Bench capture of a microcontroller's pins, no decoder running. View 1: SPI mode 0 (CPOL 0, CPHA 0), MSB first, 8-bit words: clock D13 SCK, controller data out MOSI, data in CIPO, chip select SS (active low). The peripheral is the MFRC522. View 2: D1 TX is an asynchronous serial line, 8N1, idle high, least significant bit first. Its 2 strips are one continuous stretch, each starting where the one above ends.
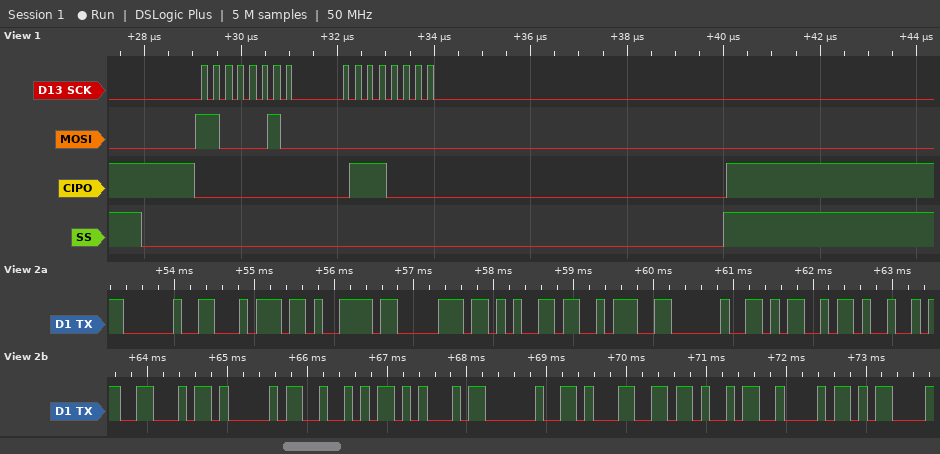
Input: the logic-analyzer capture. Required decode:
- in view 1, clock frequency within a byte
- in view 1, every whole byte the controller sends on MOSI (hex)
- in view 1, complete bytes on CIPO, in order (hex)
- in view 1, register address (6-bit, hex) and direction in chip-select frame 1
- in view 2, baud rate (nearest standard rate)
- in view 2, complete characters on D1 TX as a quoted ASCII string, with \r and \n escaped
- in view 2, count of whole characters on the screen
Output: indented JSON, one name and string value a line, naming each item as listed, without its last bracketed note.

{
  "in view 1, clock frequency within a byte": "4 MHz",
  "in view 1, every whole byte the controller sends on MOSI": "C2 00",
  "in view 1, complete bytes on CIPO, in order": "00 70",
  "in view 1, register address (6-bit, hex) and direction in chip-select frame 1": "0x21 read",
  "in view 2, baud rate": "9600 baud",
  "in view 2, complete characters on D1 TX as a quoted ASCII string, with \\r and \\n escaped": "\" type: MIFARE 1KB\\r\"",
  "in view 2, count of whole characters on the screen": "18"
}
